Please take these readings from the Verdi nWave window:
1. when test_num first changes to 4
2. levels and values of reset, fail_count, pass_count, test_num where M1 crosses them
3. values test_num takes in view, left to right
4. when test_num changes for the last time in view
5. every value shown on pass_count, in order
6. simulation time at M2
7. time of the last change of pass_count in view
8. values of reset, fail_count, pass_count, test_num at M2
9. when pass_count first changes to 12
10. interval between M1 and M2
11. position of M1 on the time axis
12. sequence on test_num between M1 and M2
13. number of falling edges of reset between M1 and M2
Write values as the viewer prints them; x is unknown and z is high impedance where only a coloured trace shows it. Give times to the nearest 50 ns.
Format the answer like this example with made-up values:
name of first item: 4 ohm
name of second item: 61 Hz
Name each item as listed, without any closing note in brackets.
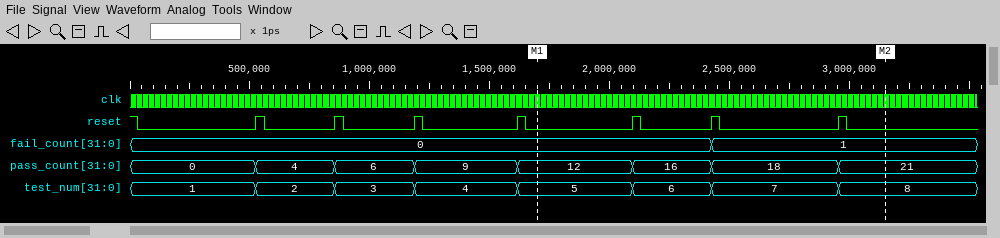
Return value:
when test_num first changes to 4: 1200 ns
levels and values of reset, fail_count, pass_count, test_num where M1 crosses them: reset=0, fail_count=0, pass_count=12, test_num=5
values test_num takes in view, left to right: 1, 2, 3, 4, 5, 6, 7, 8
when test_num changes for the last time in view: 2950 ns
every value shown on pass_count, in order: 0, 4, 6, 9, 12, 16, 18, 21
simulation time at M2: 3150 ns
time of the last change of pass_count in view: 2950 ns
values of reset, fail_count, pass_count, test_num at M2: reset=0, fail_count=1, pass_count=21, test_num=8
when pass_count first changes to 12: 1600 ns
interval between M1 and M2: 1450 ns
position of M1 on the time axis: 1700 ns
sequence on test_num between M1 and M2: 5, 6, 7, 8
number of falling edges of reset between M1 and M2: 3
